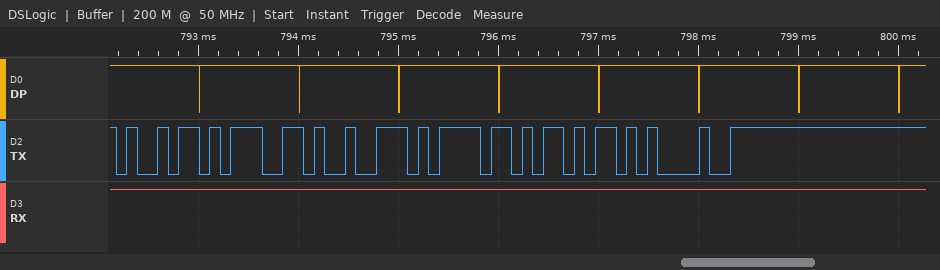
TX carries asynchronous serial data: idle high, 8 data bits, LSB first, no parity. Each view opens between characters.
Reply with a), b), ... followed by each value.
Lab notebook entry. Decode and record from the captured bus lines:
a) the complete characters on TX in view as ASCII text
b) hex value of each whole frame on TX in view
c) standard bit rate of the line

a) "igrok!"
b) 69, 67, 72, 6F, 6B, 21
c) 9600 baud
